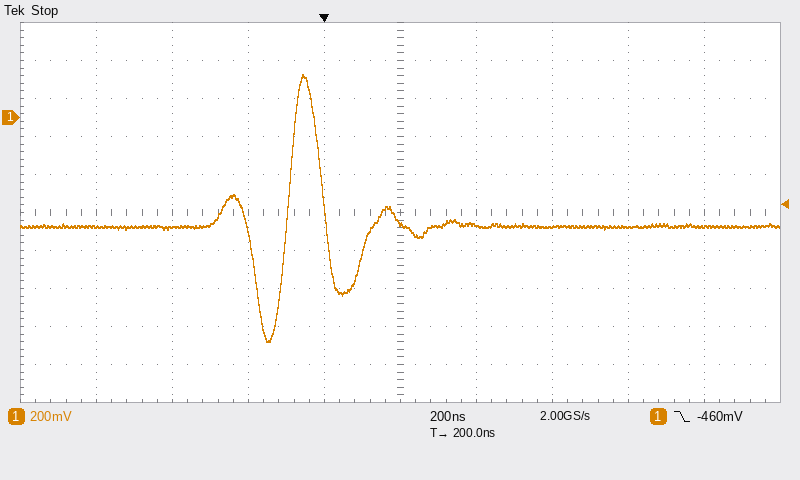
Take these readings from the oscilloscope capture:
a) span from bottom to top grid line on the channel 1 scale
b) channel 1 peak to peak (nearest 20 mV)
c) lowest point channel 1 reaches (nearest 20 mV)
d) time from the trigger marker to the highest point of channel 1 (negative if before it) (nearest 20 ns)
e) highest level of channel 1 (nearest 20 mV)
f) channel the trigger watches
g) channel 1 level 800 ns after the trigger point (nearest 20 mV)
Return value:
2 V
1.40 V
-1.18 V
-60 ns
220 mV
channel 1
-580 mV
